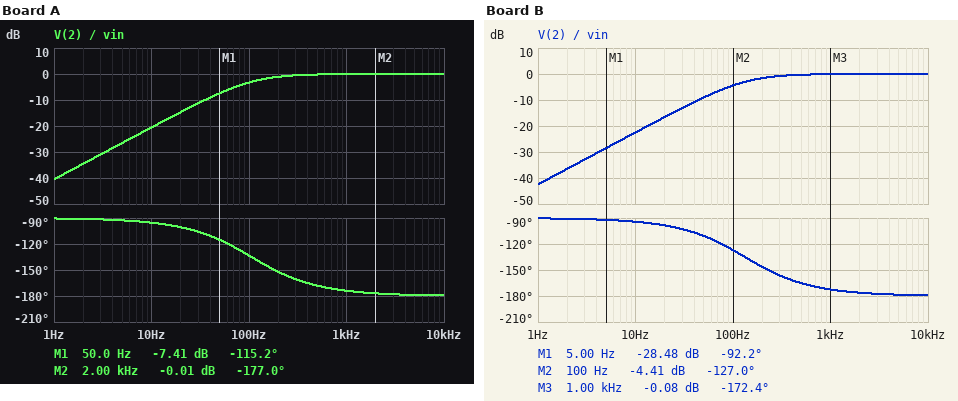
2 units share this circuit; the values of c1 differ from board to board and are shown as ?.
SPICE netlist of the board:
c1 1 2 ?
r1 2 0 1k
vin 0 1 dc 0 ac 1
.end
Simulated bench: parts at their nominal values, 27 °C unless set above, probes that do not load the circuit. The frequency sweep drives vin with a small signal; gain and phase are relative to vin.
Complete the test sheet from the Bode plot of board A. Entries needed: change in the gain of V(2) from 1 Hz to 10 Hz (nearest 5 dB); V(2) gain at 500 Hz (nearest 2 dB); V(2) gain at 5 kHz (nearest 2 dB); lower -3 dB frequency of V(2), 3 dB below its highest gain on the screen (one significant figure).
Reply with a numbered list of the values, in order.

1. 20 dB
2. 0 dB
3. 0 dB
4. 100 Hz
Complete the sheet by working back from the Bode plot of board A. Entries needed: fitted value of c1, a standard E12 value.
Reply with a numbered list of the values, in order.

1. 1.5 µF
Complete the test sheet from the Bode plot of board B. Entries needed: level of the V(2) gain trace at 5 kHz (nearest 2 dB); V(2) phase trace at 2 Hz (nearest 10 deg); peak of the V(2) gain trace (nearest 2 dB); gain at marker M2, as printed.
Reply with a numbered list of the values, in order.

1. 0 dB
2. -90 deg
3. 0 dB
4. -4.41 dB
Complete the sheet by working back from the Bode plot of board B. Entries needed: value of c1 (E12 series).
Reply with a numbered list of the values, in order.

1. 1.2 µF
